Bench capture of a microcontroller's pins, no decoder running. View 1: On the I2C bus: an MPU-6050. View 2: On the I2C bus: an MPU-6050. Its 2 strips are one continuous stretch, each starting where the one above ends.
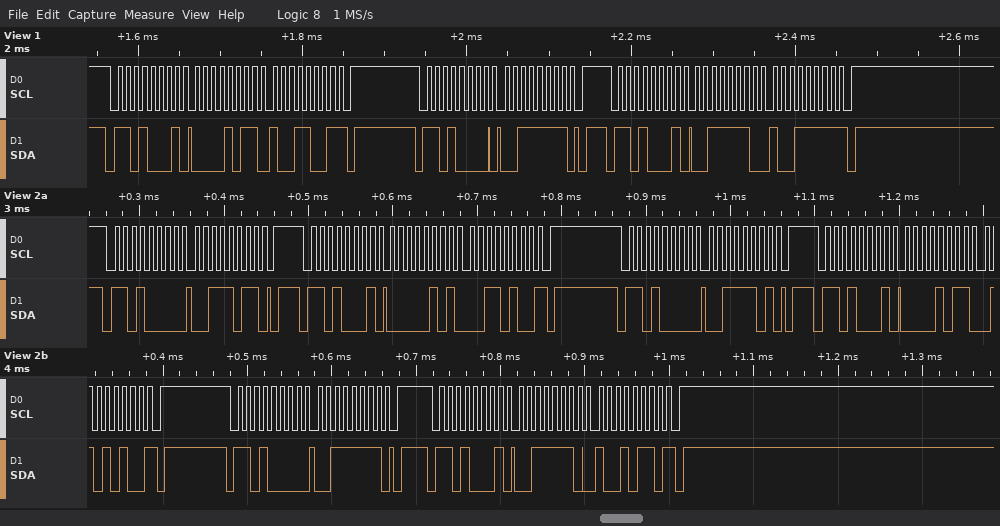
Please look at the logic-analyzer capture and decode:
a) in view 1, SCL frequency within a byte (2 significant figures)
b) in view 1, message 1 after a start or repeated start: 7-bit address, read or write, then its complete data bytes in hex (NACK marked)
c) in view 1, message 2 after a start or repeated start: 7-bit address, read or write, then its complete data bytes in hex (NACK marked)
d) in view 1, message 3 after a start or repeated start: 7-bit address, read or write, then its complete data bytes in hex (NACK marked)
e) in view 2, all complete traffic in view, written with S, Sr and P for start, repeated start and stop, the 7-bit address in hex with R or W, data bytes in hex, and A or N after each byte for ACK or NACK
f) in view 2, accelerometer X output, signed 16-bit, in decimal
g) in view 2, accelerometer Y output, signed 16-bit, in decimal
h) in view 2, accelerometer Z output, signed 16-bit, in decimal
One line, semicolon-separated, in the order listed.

100 kHz; 0x68 read: 0B 99 NACK; 0x68 write: 3F; 0x68 read: 3E 9F NACK; S 68W A 3B A P S 68R A 05 A 34 N P S 68W A 3D A P S 68R A 0B A 54 N P S 68W A 3F A P S 68R A 3E A 96 N P; 1332; 2900; 16022
